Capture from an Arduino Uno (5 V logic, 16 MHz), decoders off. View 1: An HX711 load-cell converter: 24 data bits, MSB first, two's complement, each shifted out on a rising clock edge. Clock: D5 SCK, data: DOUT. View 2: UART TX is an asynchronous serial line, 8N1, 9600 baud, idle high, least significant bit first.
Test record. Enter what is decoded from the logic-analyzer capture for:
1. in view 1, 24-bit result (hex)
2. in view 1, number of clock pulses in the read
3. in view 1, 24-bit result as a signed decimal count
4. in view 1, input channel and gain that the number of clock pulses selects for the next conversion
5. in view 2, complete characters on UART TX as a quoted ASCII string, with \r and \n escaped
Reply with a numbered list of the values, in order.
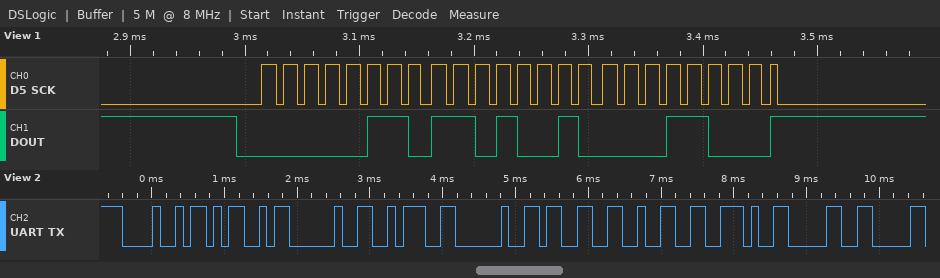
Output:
1. 0x06D218
2. 25
3. 447000
4. channel A, gain 128
5. "HM : 32.0"
